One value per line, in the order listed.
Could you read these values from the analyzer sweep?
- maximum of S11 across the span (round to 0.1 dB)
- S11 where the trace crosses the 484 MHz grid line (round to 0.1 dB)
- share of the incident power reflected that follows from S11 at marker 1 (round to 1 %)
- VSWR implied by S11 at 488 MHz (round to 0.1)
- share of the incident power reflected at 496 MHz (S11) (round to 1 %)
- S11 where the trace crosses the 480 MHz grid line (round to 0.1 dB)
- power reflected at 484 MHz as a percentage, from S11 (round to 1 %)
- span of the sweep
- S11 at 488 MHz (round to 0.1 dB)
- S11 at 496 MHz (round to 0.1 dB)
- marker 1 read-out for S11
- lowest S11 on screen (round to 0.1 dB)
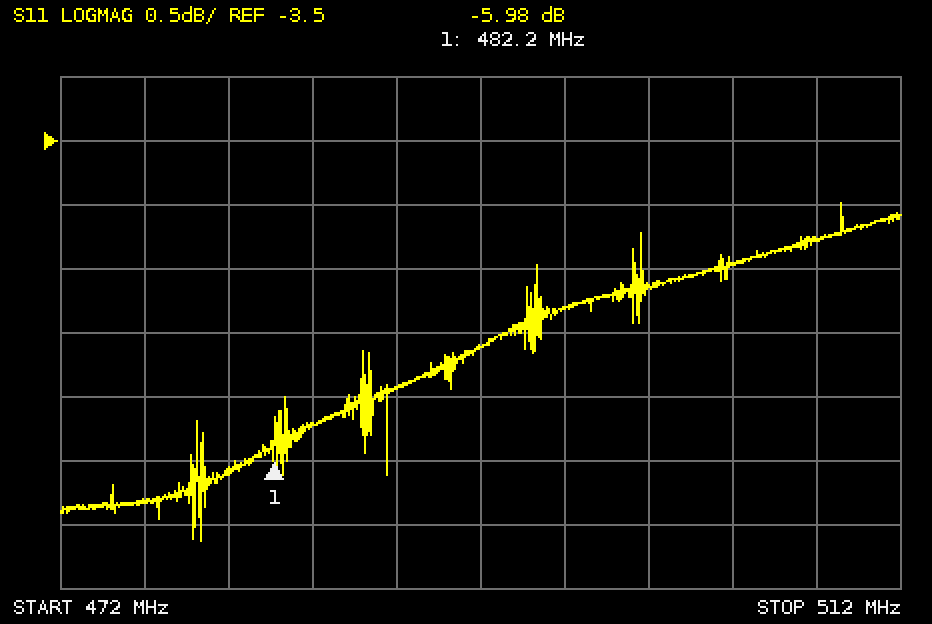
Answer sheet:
-4.0 dB
-5.7 dB
25 %
3.3
33 %
-6.1 dB
27 %
40 MHz
-5.4 dB
-4.8 dB
-5.98 dB
-6.6 dB
